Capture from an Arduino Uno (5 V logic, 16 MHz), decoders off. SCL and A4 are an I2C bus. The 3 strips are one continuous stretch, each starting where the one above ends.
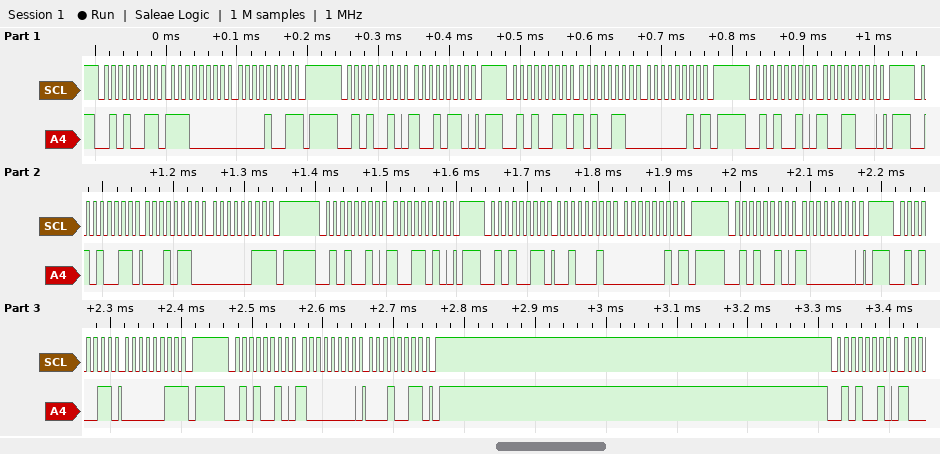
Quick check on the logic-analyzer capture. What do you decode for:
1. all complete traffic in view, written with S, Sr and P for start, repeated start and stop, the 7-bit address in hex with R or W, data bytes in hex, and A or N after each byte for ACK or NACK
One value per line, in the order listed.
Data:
S 29R A E0 A 09 N P S 29W A 96 A P S 29R A A6 A 02 N P S 29W A 98 A P S 29R A 16 A 03 N P S 29W A 9A A P S 29R A 22 A 02 N P S 29W A 80 A P S 29R A 03 N P S 29W A 80 A 13 A P S 29W A
